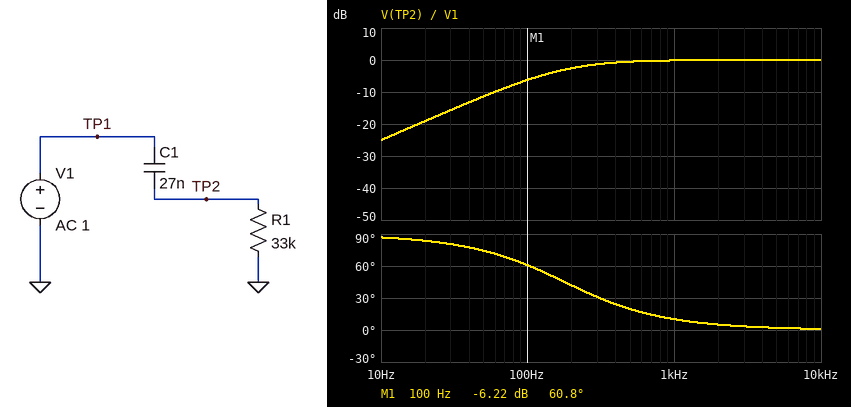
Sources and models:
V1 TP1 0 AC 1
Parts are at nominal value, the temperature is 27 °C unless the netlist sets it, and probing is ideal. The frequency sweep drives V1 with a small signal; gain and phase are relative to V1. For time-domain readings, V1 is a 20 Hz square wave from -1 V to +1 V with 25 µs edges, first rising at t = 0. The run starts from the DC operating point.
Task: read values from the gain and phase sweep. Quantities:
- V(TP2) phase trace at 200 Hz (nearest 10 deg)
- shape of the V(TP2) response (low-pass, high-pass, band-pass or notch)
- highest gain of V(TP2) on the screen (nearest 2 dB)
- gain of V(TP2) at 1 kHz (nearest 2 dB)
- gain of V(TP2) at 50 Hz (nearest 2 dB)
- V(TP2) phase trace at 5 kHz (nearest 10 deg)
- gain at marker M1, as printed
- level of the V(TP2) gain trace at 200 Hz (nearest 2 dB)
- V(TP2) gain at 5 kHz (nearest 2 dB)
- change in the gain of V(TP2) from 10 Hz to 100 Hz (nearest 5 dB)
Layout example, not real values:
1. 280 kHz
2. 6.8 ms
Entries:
1. 40 deg
2. high-pass
3. 0 dB
4. 0 dB
5. -12 dB
6. 0 deg
7. -6.22 dB
8. -2 dB
9. 0 dB
10. 20 dB
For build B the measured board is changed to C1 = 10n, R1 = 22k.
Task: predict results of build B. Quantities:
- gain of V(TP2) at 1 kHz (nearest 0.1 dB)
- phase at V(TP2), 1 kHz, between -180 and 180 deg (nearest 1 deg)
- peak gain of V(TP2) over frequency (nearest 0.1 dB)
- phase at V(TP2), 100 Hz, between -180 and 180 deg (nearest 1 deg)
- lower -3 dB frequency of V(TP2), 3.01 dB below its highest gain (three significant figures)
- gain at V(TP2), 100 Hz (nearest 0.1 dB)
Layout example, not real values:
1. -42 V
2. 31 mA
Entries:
1. -1.8 dB
2. 36 deg
3. 0 dB
4. 82 deg
5. 723 Hz
6. -17.3 dB
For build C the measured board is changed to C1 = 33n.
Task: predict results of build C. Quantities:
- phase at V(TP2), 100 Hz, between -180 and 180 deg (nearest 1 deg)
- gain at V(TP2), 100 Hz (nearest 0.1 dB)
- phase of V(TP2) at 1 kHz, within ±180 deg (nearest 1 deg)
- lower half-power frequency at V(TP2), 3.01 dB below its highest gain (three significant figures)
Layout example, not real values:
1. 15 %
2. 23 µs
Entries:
1. 56 deg
2. -5.0 dB
3. 8 deg
4. 146 Hz
